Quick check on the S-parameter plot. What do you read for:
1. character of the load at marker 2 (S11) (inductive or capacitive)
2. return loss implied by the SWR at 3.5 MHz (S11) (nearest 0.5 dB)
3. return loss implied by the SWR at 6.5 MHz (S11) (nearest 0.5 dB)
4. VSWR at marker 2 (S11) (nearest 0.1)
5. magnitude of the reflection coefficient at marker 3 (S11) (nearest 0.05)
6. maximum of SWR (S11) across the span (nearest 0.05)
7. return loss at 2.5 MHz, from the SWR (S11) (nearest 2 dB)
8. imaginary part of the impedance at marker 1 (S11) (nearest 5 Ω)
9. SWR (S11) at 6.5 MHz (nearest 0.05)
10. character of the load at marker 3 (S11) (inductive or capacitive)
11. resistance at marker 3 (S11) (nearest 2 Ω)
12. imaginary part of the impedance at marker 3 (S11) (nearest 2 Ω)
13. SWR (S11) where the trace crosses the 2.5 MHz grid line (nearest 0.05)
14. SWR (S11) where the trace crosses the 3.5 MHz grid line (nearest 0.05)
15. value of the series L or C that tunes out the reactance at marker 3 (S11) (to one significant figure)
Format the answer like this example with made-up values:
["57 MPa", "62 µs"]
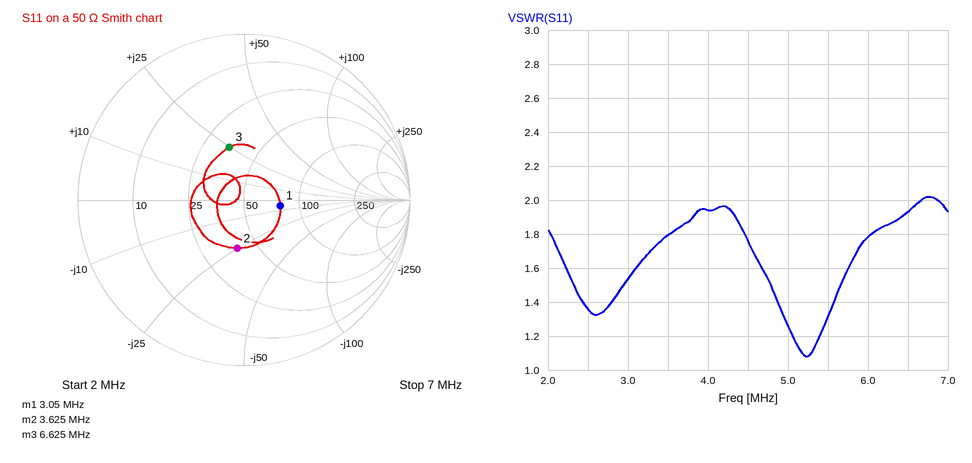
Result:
["capacitive", "11.0 dB", "10.0 dB", "1.8", "0.35", "2.00", "16 dB", "-5 Ω", "1.95", "inductive", "34 Ω", "+24 Ω", "1.35", "1.80", "1.0 nF"]
